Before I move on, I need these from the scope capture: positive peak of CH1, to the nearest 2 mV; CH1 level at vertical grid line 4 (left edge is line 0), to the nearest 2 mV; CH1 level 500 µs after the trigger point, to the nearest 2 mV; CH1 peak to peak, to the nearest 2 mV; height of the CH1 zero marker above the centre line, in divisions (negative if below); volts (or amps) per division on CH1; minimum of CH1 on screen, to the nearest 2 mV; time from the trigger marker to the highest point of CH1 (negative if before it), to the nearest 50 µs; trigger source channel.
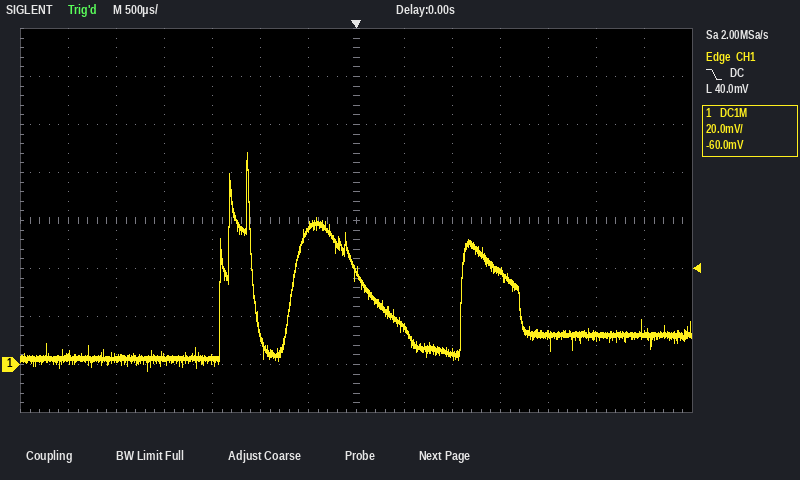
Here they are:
88 mV
2 mV
16 mV
90 mV
-3.0 div
20 mV
-2 mV
-1.15 ms
CH1
